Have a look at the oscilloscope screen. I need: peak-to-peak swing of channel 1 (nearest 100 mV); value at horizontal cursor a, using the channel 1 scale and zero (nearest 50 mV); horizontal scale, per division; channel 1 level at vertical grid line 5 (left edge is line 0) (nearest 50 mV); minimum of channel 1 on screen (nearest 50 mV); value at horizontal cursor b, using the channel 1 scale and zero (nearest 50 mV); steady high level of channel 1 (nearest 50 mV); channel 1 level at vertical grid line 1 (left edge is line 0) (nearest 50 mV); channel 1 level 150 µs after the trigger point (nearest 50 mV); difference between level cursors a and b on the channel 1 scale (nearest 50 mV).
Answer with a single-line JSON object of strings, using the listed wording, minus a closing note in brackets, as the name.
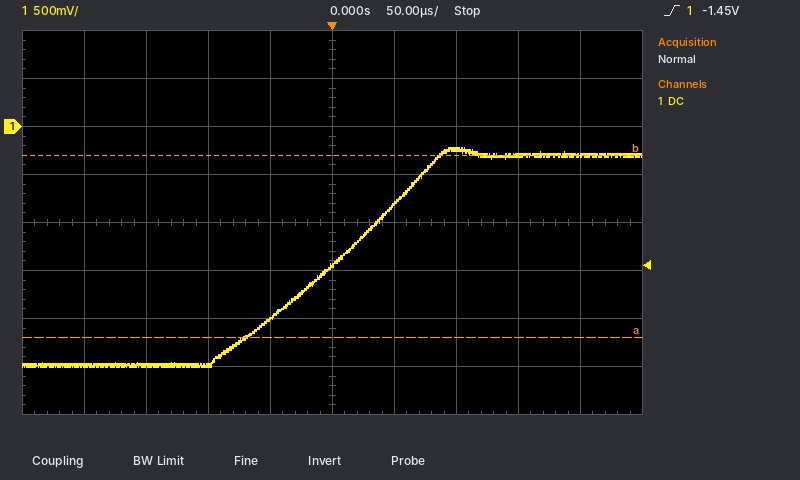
{"peak-to-peak swing of channel 1": "2.30 V", "value at horizontal cursor a, using the channel 1 scale and zero": "-2.20 V", "horizontal scale, per division": "50 µs", "channel 1 level at vertical grid line 5 (left edge is line 0)": "-1.45 V", "minimum of channel 1 on screen": "-2.50 V", "value at horizontal cursor b, using the channel 1 scale and zero": "-300 mV", "steady high level of channel 1": "-300 mV", "channel 1 level at vertical grid line 1 (left edge is line 0)": "-2.50 V", "channel 1 level 150 µs after the trigger point": "-300 mV", "difference between level cursors a and b on the channel 1 scale": "1.90 V"}
